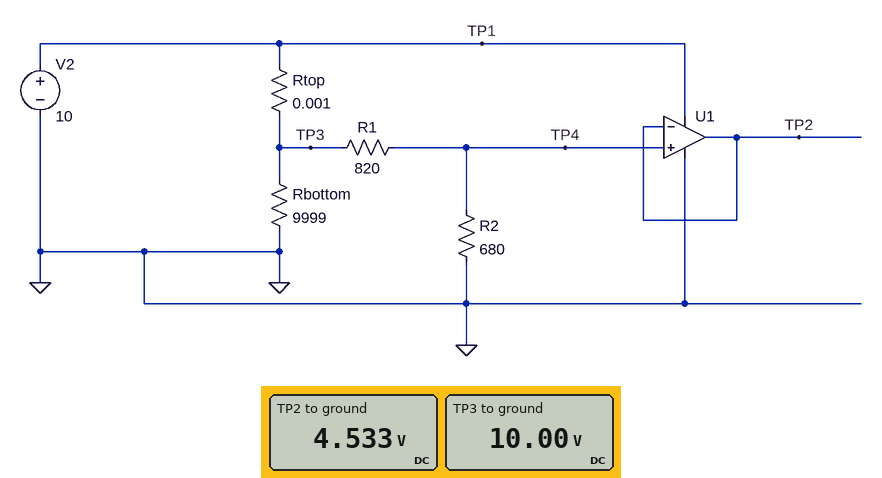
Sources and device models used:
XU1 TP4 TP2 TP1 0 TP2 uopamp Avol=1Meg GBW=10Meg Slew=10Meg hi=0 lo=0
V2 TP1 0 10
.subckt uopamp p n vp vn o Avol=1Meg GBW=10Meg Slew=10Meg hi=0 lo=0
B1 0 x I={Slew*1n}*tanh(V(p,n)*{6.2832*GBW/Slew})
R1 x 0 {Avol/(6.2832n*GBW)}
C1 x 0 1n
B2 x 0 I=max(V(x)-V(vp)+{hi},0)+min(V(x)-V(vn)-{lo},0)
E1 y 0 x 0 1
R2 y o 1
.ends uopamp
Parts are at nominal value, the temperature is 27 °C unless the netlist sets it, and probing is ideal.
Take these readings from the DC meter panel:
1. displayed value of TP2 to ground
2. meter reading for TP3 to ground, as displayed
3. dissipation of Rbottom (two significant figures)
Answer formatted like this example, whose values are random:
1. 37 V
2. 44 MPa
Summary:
1. 4.533 V
2. 10.00 V
3. 10 mW
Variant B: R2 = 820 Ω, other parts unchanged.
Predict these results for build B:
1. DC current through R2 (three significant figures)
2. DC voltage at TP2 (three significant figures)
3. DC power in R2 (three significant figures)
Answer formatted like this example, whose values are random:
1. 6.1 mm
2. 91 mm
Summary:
1. 6.10 mA
2. 5.00 V
3. 30.5 mW
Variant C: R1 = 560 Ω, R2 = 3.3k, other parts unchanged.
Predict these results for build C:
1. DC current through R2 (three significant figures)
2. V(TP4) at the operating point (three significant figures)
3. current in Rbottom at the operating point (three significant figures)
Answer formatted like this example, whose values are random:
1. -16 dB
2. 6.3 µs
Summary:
1. 2.59 mA
2. 8.55 V
3. 1.00 mA
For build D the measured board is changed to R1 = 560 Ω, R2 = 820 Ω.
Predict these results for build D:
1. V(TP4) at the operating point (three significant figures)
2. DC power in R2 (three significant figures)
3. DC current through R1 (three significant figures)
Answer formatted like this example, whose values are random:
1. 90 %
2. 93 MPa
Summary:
1. 5.94 V
2. 43.1 mW
3. 7.25 mA
